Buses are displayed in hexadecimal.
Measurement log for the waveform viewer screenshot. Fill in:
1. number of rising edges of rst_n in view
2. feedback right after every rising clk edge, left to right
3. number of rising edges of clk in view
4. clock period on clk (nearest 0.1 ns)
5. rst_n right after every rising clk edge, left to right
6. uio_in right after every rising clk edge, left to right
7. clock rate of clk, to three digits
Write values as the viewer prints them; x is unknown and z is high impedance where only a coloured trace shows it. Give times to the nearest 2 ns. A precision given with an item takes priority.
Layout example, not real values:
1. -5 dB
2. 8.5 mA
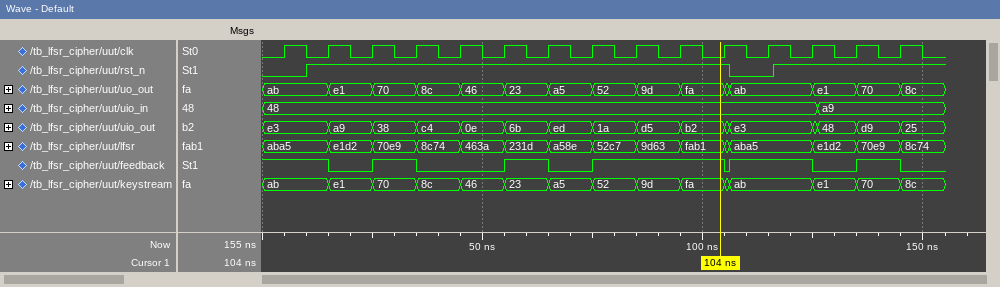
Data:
1. 2
2. 1 0 1 0 0 1 0 1 1 1 0 1 0 1 0
3. 15
4. 10 ns
5. 0 1 1 1 1 1 1 1 1 1 1 0 1 1 1
6. 48, 48, 48, 48, 48, 48, 48, 48, 48, 48, 48, 48, 48, a9, a9
7. 100 MHz
